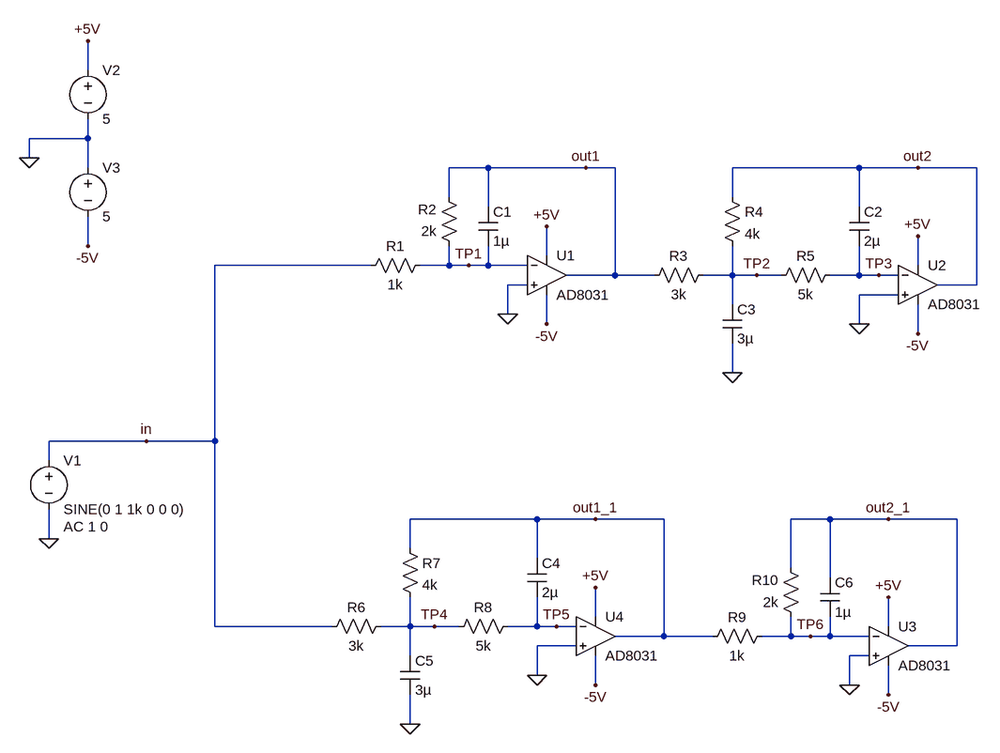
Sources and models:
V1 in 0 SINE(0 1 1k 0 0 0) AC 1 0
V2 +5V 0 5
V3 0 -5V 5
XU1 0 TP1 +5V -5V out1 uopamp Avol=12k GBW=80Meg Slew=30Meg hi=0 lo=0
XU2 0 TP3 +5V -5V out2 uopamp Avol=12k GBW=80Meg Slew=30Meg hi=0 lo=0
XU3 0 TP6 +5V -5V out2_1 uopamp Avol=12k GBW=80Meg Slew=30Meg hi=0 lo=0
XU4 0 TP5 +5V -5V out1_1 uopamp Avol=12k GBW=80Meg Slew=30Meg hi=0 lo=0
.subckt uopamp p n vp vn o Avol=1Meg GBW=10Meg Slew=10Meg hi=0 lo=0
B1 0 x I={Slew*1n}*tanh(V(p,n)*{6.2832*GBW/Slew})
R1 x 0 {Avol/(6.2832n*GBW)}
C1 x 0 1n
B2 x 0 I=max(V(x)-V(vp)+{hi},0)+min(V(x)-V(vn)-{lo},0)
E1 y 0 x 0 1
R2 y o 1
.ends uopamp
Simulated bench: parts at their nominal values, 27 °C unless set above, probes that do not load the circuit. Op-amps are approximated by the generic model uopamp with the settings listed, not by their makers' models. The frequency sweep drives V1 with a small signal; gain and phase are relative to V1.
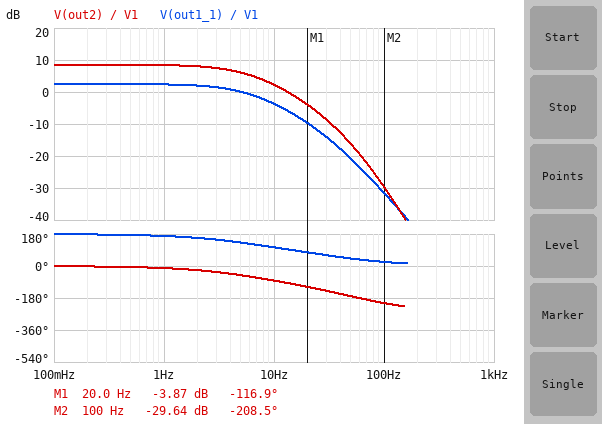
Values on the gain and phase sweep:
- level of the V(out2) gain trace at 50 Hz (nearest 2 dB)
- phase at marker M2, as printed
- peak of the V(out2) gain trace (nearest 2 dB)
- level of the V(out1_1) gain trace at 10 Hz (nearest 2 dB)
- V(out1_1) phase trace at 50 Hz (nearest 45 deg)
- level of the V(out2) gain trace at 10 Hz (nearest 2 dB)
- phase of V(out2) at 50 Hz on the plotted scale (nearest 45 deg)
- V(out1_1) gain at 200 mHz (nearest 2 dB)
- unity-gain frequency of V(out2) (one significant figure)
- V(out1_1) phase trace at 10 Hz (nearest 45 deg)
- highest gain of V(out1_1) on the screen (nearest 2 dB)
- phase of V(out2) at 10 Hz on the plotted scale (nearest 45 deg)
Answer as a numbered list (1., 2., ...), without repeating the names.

1. -16 dB
2. -208.5 deg
3. 8 dB
4. -4 dB
5. 45 deg
6. 2 dB
7. -180 deg
8. 2 dB
9. 10 Hz
10. 90 deg
11. 2 dB
12. -90 deg
